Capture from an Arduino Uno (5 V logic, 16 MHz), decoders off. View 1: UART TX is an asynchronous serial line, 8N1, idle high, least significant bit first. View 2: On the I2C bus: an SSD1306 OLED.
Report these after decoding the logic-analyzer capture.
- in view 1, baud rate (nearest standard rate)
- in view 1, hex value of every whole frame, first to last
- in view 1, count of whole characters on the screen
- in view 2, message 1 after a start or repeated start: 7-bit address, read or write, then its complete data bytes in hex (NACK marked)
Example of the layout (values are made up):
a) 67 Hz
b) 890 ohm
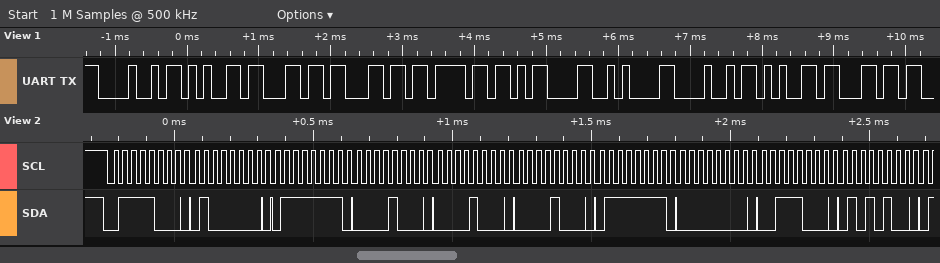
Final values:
a) 9600 baud
b) 0x48 0x65 0x6C 0x6C 0x6F 0x0D 0x0A 0x48 0x65 0x6C
c) 10
d) 0x3C write: 40 7F 08 08 08 7F 00 38 54
